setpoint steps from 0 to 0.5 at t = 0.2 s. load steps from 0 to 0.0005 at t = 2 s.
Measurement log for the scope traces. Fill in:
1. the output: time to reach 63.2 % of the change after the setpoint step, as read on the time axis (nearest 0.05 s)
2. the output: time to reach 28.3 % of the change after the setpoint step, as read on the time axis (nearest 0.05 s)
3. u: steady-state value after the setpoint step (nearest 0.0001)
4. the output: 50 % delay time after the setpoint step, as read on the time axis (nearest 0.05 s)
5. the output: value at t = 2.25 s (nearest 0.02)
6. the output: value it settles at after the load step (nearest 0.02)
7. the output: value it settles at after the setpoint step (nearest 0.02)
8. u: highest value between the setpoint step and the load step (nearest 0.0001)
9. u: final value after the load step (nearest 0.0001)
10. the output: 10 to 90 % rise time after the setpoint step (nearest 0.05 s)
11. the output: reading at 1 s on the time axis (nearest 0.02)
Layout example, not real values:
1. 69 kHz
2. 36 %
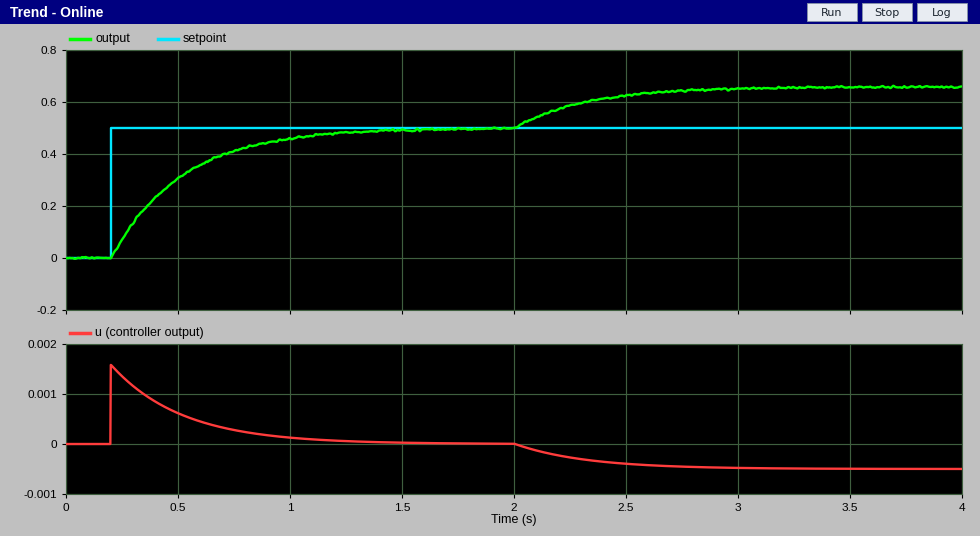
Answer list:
1. 0.50 s
2. 0.30 s
3. 0.0000
4. 0.40 s
5. 0.58
6. 0.66
7. 0.50
8. 0.0016
9. -0.0005
10. 0.70 s
11. 0.46
